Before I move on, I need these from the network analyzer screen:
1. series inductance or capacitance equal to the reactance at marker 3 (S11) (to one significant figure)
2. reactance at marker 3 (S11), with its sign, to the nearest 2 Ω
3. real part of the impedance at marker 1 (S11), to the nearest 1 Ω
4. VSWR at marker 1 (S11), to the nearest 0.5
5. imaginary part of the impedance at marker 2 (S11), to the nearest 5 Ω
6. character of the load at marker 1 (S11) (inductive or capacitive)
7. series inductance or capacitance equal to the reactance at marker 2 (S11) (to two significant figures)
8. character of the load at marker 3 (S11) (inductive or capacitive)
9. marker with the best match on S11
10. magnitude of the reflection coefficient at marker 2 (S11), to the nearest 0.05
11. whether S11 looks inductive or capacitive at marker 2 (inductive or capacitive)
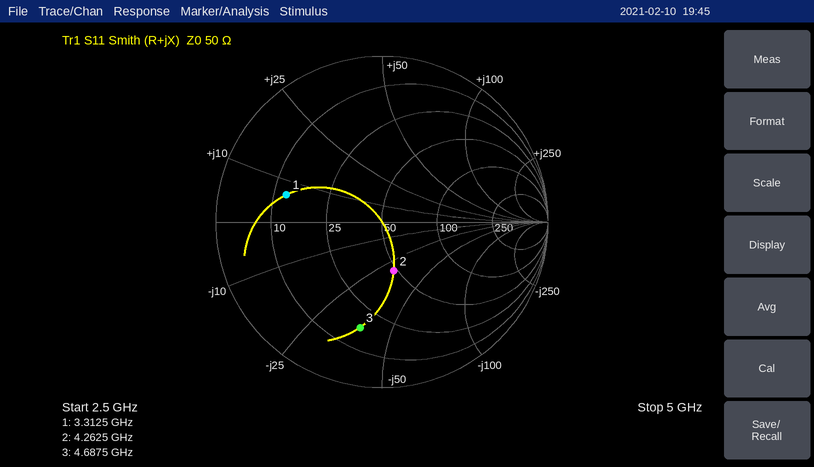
900 fF
-38 Ω
13 Ω
4.0
-30 Ω
inductive
1.2 pF
capacitive
marker 2
0.30
capacitive
